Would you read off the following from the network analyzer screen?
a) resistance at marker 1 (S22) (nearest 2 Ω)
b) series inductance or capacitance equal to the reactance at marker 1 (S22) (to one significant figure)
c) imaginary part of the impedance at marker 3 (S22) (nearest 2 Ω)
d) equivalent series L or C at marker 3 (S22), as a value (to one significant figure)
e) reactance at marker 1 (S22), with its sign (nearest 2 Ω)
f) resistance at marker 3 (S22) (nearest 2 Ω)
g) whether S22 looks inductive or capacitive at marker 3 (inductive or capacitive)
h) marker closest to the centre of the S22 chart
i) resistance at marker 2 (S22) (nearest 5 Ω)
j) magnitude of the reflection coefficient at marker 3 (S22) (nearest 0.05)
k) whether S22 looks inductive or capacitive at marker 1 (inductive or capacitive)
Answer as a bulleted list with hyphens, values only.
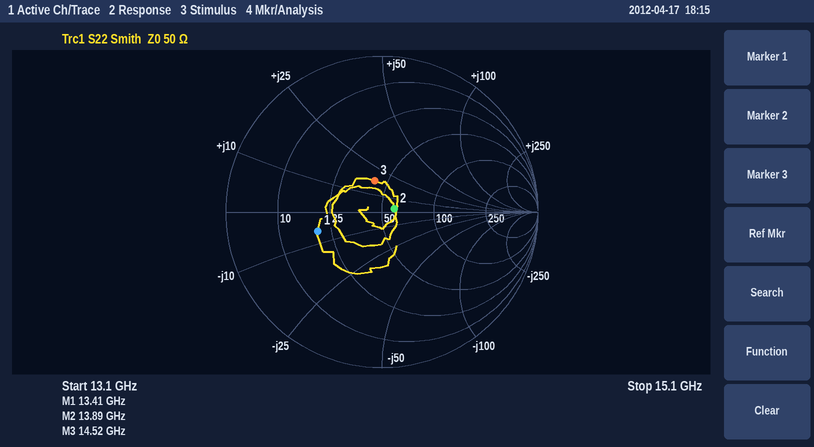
- 20 Ω
- 2 pF
- +18 Ω
- 200 pH
- -6 Ω
- 42 Ω
- inductive
- marker 2
- 60 Ω
- 0.20
- capacitive
